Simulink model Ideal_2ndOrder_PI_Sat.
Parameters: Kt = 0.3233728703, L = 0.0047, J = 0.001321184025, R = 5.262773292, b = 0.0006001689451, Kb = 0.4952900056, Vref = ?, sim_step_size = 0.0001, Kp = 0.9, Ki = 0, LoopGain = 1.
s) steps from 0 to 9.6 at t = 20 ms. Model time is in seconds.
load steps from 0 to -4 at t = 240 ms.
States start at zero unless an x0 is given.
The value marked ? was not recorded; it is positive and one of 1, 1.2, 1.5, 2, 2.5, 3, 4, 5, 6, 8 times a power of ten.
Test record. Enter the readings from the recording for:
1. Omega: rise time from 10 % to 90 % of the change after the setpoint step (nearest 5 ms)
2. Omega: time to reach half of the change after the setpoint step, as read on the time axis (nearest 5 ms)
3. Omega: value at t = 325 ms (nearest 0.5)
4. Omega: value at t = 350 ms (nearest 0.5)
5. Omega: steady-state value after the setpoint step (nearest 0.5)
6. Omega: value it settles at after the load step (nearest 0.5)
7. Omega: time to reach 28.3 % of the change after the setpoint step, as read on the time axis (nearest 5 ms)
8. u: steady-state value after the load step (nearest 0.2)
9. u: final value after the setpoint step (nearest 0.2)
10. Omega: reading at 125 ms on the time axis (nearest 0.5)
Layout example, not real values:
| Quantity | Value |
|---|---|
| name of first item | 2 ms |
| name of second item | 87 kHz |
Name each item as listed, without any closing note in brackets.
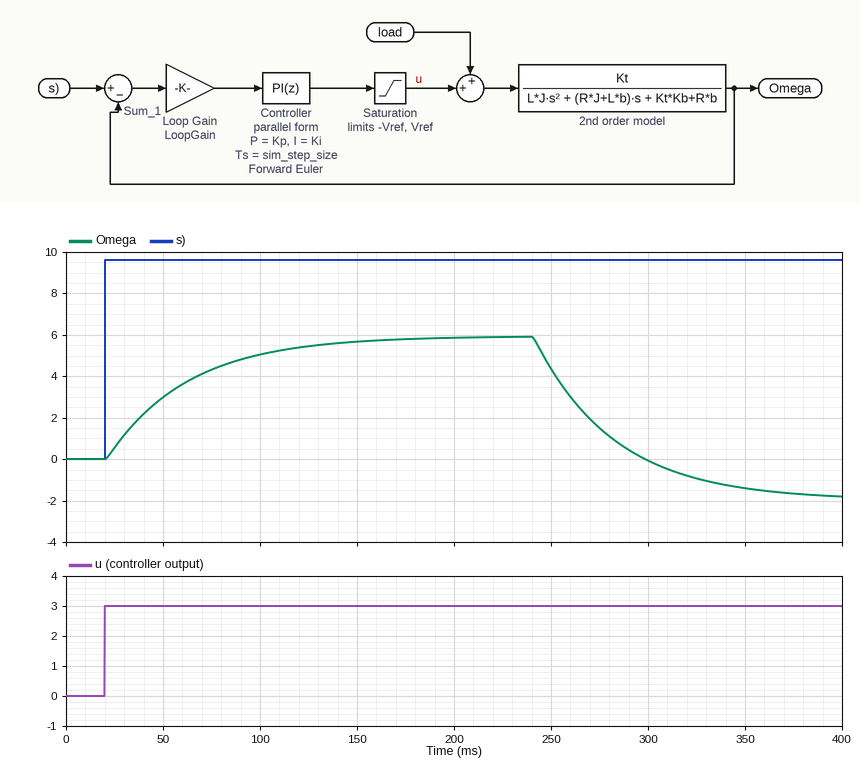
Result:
| Quantity | Value |
|---|---|
| Omega: rise time from 10 % to 90 % of the change after the setpoint step | 90 ms |
| Omega: time to reach half of the change after the setpoint step, as read on the time axis | 50 ms |
| Omega: value at t = 325 ms | -1.0 |
| Omega: value at t = 350 ms | -1.5 |
| Omega: steady-state value after the setpoint step | 6.0 |
| Omega: value it settles at after the load step | -2.0 |
| Omega: time to reach 28.3 % of the change after the setpoint step, as read on the time axis | 35 ms |
| u: steady-state value after the load step | 3.0 |
| u: final value after the setpoint step | 3.0 |
| Omega: reading at 125 ms on the time axis | 5.5 |
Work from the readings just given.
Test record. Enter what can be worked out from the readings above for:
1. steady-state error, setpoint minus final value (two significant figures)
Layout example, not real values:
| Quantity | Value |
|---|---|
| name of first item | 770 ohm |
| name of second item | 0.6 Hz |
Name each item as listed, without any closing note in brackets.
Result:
| Quantity | Value |
|---|---|
| steady-state error, setpoint minus final value | 3.6 |
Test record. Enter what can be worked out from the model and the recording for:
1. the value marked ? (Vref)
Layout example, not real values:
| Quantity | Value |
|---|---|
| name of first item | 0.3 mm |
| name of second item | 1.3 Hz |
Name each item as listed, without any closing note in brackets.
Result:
| Quantity | Value |
|---|---|
| the value marked ? | 3 |
